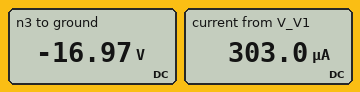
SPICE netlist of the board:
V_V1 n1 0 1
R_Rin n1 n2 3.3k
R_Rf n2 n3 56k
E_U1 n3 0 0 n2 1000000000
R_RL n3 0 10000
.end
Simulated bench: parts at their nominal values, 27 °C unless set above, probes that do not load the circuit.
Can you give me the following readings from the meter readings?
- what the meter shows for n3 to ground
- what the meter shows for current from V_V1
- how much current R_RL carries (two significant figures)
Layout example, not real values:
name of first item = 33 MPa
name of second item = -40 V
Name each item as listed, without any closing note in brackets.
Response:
what the meter shows for n3 to ground = -16.97 V
what the meter shows for current from V_V1 = 303.0 µA
how much current R_RL carries = 1.7 mA
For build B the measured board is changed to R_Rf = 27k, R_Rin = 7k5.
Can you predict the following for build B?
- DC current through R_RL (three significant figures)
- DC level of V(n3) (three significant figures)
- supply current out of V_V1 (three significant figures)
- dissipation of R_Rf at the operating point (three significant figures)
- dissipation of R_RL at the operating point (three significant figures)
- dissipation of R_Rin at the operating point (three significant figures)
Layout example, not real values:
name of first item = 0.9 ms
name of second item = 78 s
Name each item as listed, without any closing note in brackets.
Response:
DC current through R_RL = 360 µA
DC level of V(n3) = -3.60 V
supply current out of V_V1 = 133 µA
dissipation of R_Rf at the operating point = 480 µW
dissipation of R_RL at the operating point = 1.30 mW
dissipation of R_Rin at the operating point = 133 µW
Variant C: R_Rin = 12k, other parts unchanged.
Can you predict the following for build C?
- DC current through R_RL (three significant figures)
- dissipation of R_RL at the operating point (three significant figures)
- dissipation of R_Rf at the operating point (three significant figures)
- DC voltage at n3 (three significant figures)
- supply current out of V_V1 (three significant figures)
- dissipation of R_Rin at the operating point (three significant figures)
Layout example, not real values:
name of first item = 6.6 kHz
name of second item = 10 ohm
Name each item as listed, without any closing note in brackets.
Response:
DC current through R_RL = 467 µA
dissipation of R_RL at the operating point = 2.18 mW
dissipation of R_Rf at the operating point = 389 µW
DC voltage at n3 = -4.67 V
supply current out of V_V1 = 83.3 µA
dissipation of R_Rin at the operating point = 83.3 µW
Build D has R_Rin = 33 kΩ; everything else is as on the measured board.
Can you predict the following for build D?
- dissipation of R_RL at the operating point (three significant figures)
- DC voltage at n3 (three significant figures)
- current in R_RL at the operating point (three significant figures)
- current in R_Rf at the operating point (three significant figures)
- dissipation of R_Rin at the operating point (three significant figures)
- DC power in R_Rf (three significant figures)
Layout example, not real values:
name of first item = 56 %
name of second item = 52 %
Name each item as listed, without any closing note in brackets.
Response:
dissipation of R_RL at the operating point = 288 µW
DC voltage at n3 = -1.70 V
current in R_RL at the operating point = 170 µA
current in R_Rf at the operating point = 30.3 µA
dissipation of R_Rin at the operating point = 30.3 µW
DC power in R_Rf = 51.4 µW
